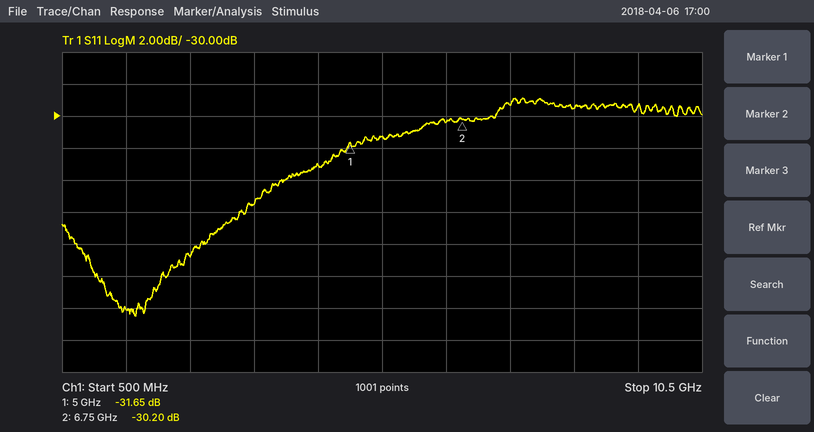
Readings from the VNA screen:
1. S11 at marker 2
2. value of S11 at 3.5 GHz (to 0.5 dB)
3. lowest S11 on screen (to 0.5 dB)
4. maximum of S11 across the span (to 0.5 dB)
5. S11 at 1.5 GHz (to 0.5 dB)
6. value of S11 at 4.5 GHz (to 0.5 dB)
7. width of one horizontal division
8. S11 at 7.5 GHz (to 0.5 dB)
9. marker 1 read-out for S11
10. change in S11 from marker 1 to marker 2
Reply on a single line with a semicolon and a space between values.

-30.20 dB; -35.5 dB; -42.5 dB; -29.0 dB; -42.0 dB; -33.0 dB; 1 GHz; -29.5 dB; -31.65 dB; 1.45 dB
